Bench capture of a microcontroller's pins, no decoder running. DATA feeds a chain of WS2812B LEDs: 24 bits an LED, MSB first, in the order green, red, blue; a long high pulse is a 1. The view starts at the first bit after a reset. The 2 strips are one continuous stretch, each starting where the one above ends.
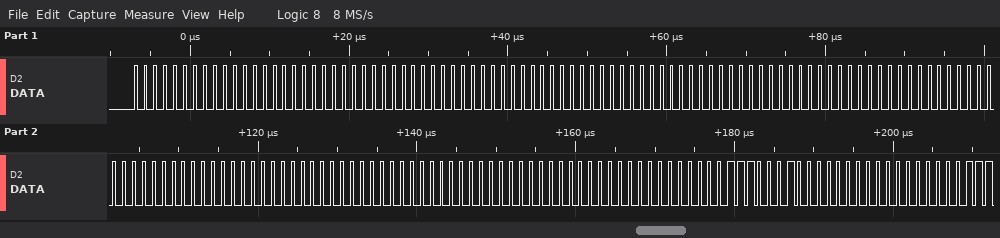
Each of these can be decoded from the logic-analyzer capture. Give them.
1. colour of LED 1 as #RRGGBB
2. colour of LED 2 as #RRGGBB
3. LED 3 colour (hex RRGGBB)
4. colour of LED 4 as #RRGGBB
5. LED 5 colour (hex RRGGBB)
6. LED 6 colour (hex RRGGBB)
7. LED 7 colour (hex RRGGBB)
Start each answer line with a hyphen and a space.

- #000000
- #000000
- #000000
- #000000
- #000000
- #000000
- #100700
